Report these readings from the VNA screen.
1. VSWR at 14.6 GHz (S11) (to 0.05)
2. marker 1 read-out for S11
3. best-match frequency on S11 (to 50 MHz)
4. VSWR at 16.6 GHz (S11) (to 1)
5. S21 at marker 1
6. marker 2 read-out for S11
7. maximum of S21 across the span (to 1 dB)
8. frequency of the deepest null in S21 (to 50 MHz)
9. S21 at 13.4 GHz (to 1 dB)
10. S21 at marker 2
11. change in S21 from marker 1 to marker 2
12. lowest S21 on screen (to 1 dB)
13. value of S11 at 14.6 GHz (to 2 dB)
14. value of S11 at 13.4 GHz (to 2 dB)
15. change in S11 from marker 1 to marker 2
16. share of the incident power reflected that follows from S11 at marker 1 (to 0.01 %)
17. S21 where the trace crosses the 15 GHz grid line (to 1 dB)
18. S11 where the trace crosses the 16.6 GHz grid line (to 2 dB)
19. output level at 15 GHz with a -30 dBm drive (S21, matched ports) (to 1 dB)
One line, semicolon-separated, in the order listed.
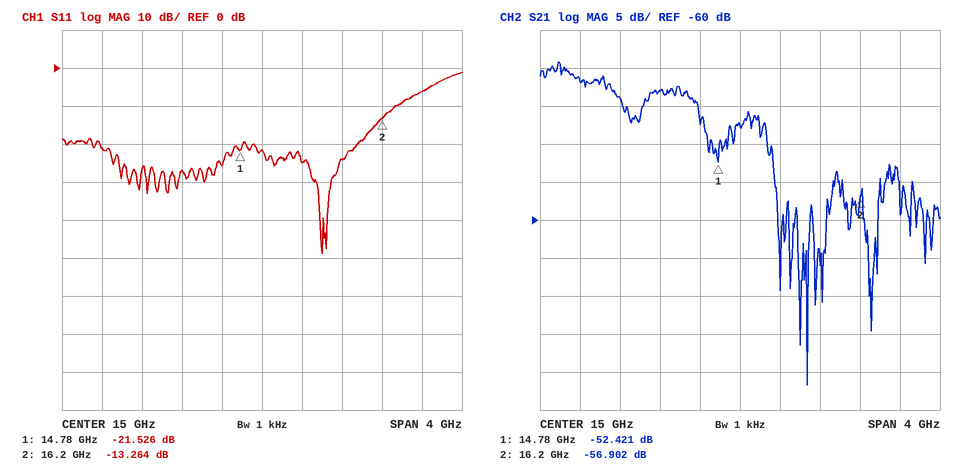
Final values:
1.10; -21.526 dB; 15.60 GHz; 3; -52.421 dB; -13.264 dB; -39 dB; 15.65 GHz; -42 dB; -56.902 dB; -4.481 dB; -82 dB; -26 dB; -22 dB; 8.262 dB; 0.70 %; -48 dB; -6 dB; -78 dBm
